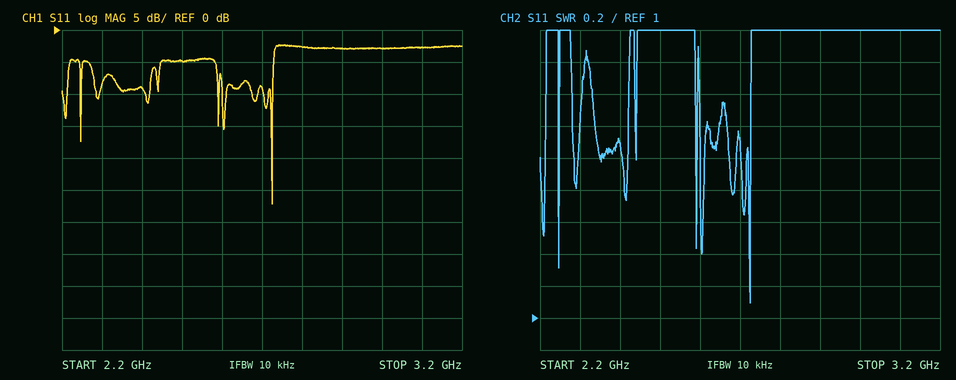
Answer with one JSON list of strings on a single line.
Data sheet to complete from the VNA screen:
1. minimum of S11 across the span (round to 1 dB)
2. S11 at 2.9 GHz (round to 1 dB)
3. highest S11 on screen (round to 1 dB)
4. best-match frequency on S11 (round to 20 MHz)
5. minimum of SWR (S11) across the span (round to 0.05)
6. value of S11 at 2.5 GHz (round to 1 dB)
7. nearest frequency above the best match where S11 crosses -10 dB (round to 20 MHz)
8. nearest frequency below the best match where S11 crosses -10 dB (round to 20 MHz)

["-27 dB", "-3 dB", "-2 dB", "2.72 GHz", "1.10", "-5 dB", "2.72 GHz", "2.72 GHz"]
